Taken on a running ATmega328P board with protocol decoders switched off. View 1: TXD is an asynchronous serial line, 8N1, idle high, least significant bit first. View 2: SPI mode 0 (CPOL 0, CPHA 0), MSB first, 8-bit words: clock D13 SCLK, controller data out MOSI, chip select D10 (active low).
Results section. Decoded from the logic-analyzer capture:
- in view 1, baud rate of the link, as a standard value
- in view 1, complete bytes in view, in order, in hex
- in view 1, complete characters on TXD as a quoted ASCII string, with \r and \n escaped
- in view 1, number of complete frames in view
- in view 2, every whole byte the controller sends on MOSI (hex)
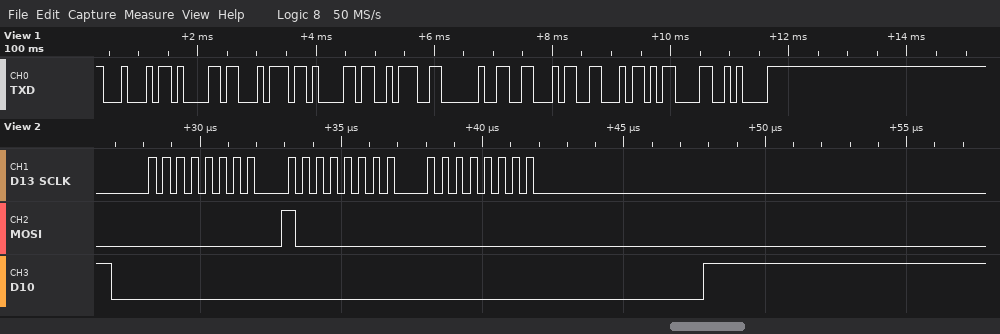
9600 baud
0x44 0x61 0x74 0x61 0x3A 0x20 0x46 0x46 0x0D 0x0A
"Data: FF\r\n"
10
00 80 00
